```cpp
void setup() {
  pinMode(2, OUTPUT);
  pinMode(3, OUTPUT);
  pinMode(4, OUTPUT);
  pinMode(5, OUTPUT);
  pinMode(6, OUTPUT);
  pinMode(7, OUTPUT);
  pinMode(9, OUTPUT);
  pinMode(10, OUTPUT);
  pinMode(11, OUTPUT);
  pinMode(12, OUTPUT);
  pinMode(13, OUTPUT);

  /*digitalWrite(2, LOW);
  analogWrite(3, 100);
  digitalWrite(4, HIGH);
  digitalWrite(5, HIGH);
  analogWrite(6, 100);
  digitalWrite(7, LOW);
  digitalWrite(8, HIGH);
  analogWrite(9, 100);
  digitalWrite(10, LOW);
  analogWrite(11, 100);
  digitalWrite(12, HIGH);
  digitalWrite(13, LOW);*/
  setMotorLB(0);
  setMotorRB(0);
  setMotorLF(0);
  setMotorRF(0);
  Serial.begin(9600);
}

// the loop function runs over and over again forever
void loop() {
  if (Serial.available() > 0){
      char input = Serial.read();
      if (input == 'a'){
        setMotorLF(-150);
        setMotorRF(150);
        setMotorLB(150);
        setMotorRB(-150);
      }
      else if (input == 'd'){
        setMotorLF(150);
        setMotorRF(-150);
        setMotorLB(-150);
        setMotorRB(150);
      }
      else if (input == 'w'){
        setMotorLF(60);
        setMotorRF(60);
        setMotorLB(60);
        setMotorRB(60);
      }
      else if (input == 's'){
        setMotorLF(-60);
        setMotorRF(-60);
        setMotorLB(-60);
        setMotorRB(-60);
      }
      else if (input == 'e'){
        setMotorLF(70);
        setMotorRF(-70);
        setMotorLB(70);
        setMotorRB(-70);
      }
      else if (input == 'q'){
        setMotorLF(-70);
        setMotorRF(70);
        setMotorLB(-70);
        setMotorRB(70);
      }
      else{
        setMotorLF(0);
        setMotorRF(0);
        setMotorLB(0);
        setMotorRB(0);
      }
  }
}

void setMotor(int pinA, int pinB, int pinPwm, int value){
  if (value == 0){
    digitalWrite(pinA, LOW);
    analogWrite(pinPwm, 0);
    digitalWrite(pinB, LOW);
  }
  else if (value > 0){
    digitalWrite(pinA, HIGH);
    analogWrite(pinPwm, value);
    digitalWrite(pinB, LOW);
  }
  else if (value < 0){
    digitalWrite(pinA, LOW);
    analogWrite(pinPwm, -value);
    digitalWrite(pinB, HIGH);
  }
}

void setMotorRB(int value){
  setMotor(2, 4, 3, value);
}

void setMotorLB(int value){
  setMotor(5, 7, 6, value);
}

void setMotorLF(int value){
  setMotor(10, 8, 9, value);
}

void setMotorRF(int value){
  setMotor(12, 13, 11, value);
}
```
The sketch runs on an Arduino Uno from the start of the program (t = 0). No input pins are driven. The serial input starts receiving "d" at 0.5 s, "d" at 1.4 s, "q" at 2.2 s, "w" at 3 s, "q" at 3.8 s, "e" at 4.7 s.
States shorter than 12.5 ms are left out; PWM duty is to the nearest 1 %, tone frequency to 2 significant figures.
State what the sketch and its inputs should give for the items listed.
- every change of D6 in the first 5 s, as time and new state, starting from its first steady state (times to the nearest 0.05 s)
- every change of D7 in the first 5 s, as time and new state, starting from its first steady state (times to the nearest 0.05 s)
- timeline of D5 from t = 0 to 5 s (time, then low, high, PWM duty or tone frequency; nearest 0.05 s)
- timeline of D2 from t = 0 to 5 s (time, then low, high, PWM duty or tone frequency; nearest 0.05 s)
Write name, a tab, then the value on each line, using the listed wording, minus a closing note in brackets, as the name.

every change of D6 in the first 5 s, as time and new state, starting from its first steady state	0 s low; 0.5 s PWM 59 %; 2.2 s PWM 28 %; 3 s PWM 24 %; 3.8 s PWM 28 %
every change of D7 in the first 5 s, as time and new state, starting from its first steady state	0 s low; 0.5 s high; 3 s low; 3.8 s high; 4.7 s low
timeline of D5 from t = 0 to 5 s	0 s low; 3 s high; 3.8 s low; 4.7 s high
timeline of D2 from t = 0 to 5 s	0 s low; 0.5 s high; 4.7 s low
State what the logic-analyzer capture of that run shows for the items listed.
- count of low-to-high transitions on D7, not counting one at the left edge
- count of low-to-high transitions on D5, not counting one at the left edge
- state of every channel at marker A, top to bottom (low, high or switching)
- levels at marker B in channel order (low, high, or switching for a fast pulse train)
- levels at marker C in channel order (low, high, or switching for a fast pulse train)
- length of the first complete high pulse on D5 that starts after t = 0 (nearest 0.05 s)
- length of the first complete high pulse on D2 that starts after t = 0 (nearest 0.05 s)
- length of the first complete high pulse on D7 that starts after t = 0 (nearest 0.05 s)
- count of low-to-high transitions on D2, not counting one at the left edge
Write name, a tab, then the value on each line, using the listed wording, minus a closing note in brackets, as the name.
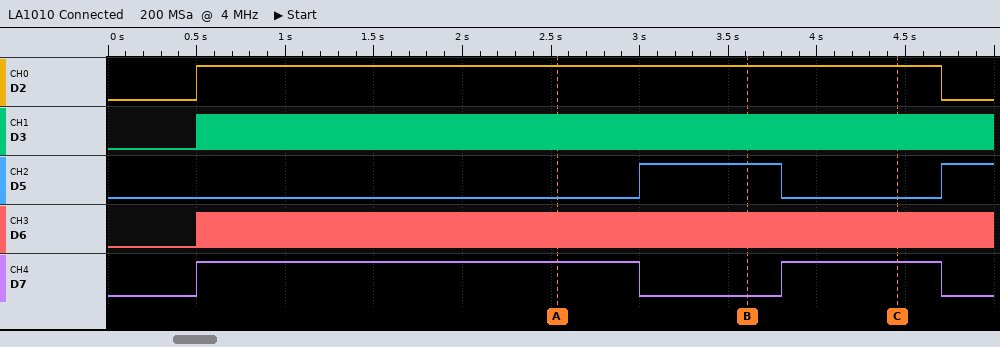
count of low-to-high transitions on D7, not counting one at the left edge	2
count of low-to-high transitions on D5, not counting one at the left edge	2
state of every channel at marker A, top to bottom	D2 high, D3 switching, D5 low, D6 switching, D7 high
levels at marker B in channel order	D2 high, D3 switching, D5 high, D6 switching, D7 low
levels at marker C in channel order	D2 high, D3 switching, D5 low, D6 switching, D7 high
length of the first complete high pulse on D5 that starts after t = 0	0.80 s
length of the first complete high pulse on D2 that starts after t = 0	4.20 s
length of the first complete high pulse on D7 that starts after t = 0	2.50 s
count of low-to-high transitions on D2, not counting one at the left edge	1
